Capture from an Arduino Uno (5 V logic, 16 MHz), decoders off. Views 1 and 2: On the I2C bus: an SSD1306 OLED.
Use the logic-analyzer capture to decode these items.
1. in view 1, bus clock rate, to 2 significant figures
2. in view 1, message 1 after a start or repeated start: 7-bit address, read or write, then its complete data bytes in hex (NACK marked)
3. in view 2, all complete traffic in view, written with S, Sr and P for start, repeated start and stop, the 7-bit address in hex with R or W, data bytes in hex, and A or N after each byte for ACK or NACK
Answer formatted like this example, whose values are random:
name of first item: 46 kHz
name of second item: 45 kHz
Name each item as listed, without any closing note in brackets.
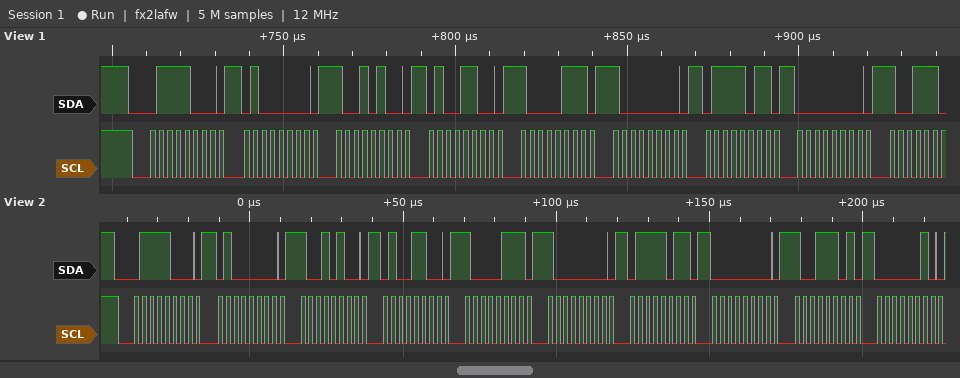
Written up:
in view 1, bus clock rate, to 2 significant figures: 400 kHz
in view 1, message 1 after a start or repeated start: 7-bit address, read or write, then its complete data bytes in hex: 0x3C write: 40 94 4C 87 80 7B 00
in view 2, all complete traffic in view, written with S, Sr and P for start, repeated start and stop, the 7-bit address in hex with R or W, data bytes in hex, and A or N after each byte for ACK or NACK: S 3CW A 40 A 94 A 4C A 87 A 80 A 7B A 00 A 9D A 02 A
